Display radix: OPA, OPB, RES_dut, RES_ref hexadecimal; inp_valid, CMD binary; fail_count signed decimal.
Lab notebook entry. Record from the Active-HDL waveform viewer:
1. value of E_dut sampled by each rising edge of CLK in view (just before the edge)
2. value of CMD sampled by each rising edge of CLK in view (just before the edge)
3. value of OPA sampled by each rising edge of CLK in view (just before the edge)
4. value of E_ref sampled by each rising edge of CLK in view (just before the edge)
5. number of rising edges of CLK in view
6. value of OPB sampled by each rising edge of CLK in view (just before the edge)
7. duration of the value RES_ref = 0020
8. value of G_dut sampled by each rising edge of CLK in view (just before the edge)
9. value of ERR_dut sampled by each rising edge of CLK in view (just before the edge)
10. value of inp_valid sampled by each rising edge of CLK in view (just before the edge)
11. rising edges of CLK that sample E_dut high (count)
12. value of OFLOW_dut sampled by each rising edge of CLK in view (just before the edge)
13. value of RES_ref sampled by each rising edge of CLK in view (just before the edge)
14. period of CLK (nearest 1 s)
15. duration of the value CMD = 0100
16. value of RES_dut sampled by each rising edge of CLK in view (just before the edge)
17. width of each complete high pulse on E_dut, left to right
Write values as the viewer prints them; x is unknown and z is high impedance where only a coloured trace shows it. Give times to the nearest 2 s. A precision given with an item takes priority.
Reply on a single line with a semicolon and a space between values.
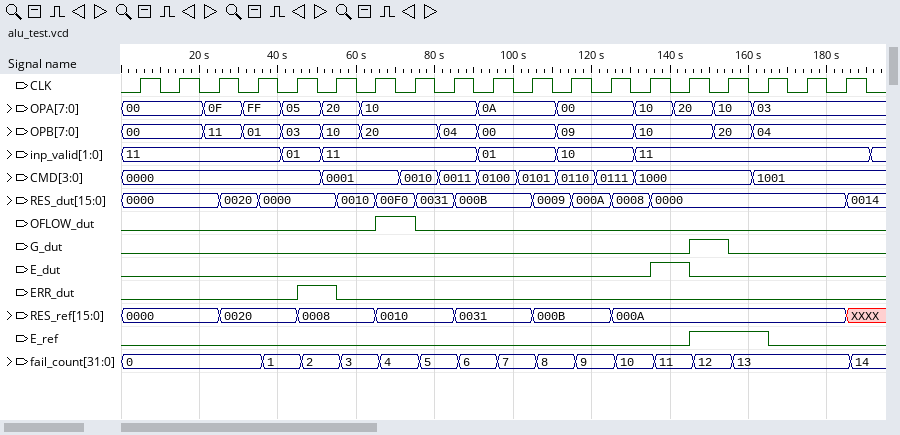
0 0 0 0 0 0 0 0 0 0 0 0 0 0 1 0 0 0 0; 0000, 0000, 0000, 0000, 0000, 0001, 0001, 0010, 0011, 0100, 0101, 0110, 0111, 1000, 1000, 1000, 1001, 1001, 1001; 00, 00, 0F, FF, 05, 20, 10, 10, 10, 0A, 0A, 00, 00, 10, 20, 10, 03, 03, 03; 0 0 0 0 0 0 0 0 0 0 0 0 0 0 0 1 1 0 0; 19; 00, 00, 11, 01, 03, 10, 20, 20, 04, 00, 00, 09, 09, 10, 10, 20, 04, 04, 04; 20 s; 0 0 0 0 0 0 0 0 0 0 0 0 0 0 0 1 0 0 0; 0 0 0 0 0 1 0 0 0 0 0 0 0 0 0 0 0 0 0; 11, 11, 11, 11, 01, 11, 11, 11, 11, 01, 01, 10, 10, 11, 11, 11, 11, 11, 11; 1; 0 0 0 0 0 0 0 1 0 0 0 0 0 0 0 0 0 0 0; 0000, 0000, 0000, 0020, 0020, 0008, 0008, 0010, 0010, 0031, 0031, 000B, 000B, 000A, 000A, 000A, 000A, 000A, 000A; 10 s; 10 s; 0000, 0000, 0000, 0020, 0000, 0000, 0010, 00F0, 0031, 000B, 000B, 0009, 000A, 0008, 0000, 0000, 0000, 0000, 0000; 10 s
